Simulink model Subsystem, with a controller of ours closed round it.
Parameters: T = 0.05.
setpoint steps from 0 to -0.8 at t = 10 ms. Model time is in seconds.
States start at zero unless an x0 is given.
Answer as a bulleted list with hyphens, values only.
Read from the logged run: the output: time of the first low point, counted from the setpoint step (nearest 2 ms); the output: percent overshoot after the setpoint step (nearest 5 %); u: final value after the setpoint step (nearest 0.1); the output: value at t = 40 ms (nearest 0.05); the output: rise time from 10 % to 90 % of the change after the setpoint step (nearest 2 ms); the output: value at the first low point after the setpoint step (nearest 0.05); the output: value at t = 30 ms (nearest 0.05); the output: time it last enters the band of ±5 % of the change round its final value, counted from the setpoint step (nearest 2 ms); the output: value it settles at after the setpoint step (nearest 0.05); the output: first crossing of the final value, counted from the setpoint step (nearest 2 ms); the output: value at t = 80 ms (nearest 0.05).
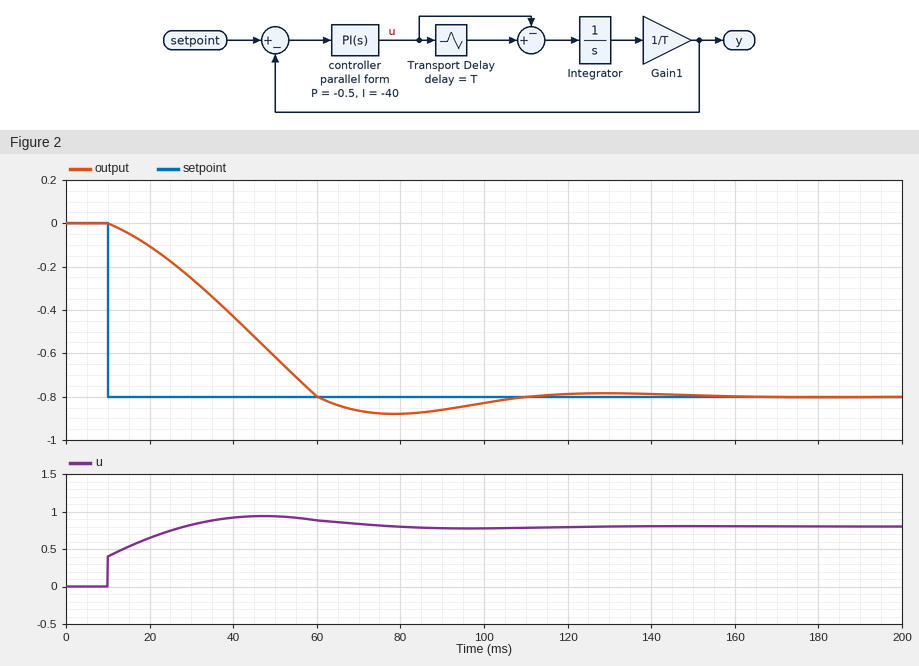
- 68 ms
- 10 %
- 0.8
- -0.45
- 38 ms
- -0.90
- -0.25
- 86 ms
- -0.80
- 50 ms
- -0.90
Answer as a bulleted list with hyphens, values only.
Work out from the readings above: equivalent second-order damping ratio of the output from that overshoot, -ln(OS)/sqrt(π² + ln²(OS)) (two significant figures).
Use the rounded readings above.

- 0.59
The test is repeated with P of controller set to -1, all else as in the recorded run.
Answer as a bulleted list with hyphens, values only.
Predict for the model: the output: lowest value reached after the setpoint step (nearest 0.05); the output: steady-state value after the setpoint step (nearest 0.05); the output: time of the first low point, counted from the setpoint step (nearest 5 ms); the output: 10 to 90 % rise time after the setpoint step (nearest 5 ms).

- -0.85
- -0.80
- 50 ms
- 35 ms
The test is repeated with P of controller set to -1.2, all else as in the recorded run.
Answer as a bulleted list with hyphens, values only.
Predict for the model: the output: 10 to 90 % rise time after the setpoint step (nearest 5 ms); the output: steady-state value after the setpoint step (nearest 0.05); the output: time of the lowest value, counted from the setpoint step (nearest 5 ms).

- 35 ms
- -0.80
- 50 ms
